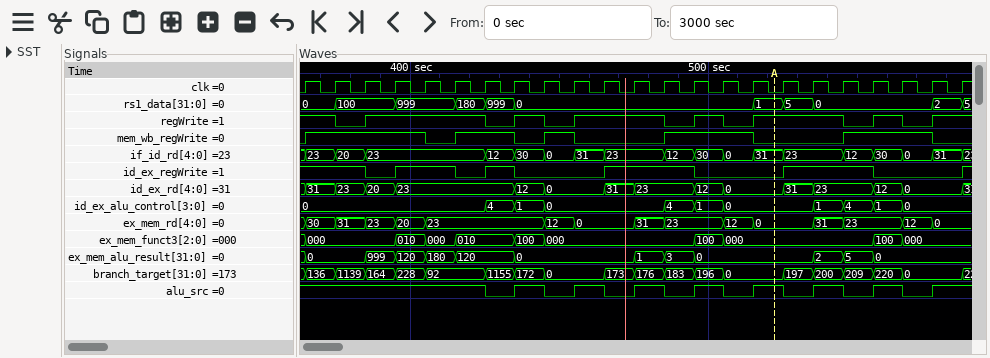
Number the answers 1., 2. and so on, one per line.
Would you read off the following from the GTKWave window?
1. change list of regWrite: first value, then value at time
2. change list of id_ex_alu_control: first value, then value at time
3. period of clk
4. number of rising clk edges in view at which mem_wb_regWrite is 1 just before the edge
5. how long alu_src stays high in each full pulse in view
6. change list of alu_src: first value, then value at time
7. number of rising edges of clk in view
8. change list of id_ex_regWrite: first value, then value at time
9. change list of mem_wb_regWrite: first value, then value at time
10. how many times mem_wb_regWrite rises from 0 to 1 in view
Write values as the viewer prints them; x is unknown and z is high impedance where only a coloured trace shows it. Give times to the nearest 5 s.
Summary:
1. 1, 0 at 375 s, 1 at 385 s, 0 at 425 s, 1 at 435 s, 0 at 445 s, 1 at 455 s, 0 at 485 s, 1 at 495 s, 0 at 505 s, 1 at 515 s, 0 at 545 s, 1 at 555 s, 0 at 565 s, 1 at 575 s
2. 0, 4 at 425 s, 1 at 435 s, 0 at 445 s, 4 at 485 s, 1 at 495 s, 0 at 505 s, 1 at 535 s, 4 at 545 s, 1 at 555 s, 0 at 565 s
3. 10 s
4. 13
5. 10 s, 10 s, 10 s, 10 s, 10 s, 10 s, 10 s
6. 1, 0 at 425 s, 1 at 435 s, 0 at 445 s, 1 at 455 s, 0 at 465 s, 1 at 475 s, 0 at 485 s, 1 at 495 s, 0 at 505 s, 1 at 515 s, 0 at 525 s, 1 at 535 s, 0 at 545 s, 1 at 555 s, 0 at 565 s, 1 at 575 s
7. 23
8. 1, 0 at 385 s, 1 at 395 s, 0 at 415 s, 1 at 425 s, 0 at 435 s, 1 at 465 s, 0 at 495 s, 1 at 525 s, 0 at 555 s, 1 at 585 s
9. 0, 1 at 365 s, 0 at 405 s, 1 at 415 s, 0 at 435 s, 1 at 445 s, 0 at 455 s, 1 at 485 s, 0 at 515 s, 1 at 545 s, 0 at 575 s
10. 5
